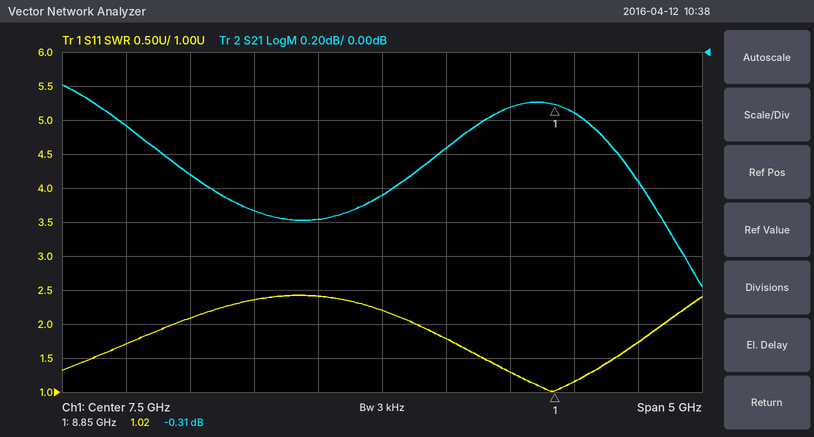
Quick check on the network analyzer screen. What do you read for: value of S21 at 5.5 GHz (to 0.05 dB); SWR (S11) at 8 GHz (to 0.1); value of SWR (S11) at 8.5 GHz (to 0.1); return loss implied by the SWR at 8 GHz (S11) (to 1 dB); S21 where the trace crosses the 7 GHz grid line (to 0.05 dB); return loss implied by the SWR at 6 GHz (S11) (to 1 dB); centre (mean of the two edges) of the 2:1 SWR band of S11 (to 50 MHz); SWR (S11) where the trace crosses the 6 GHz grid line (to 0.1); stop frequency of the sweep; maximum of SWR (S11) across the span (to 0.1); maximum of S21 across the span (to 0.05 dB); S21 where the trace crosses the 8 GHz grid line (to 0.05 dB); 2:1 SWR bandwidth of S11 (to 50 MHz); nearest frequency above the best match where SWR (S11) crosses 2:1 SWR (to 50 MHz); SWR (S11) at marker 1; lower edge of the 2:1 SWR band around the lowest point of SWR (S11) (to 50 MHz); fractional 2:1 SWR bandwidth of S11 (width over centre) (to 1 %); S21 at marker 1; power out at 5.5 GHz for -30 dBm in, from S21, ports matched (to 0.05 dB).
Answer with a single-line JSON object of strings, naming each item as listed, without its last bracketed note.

{"value of S21 at 5.5 GHz": "-0.45 dB", "SWR (S11) at 8 GHz": "1.8", "value of SWR (S11) at 8.5 GHz": "1.3", "return loss implied by the SWR at 8 GHz (S11)": "11 dB", "S21 where the trace crosses the 7 GHz grid line": "-1.00 dB", "return loss implied by the SWR at 6 GHz (S11)": "9 dB", "centre (mean of the two edges) of the 2:1 SWR band of S11": "8.75 GHz", "SWR (S11) where the trace crosses the 6 GHz grid line": "2.1", "stop frequency of the sweep": "10 GHz", "maximum of SWR (S11) across the span": "2.4", "maximum of S21 across the span": "-0.20 dB", "S21 where the trace crosses the 8 GHz grid line": "-0.55 dB", "2:1 SWR bandwidth of S11": "1.95 GHz", "nearest frequency above the best match where SWR (S11) crosses 2:1 SWR": "9.70 GHz", "SWR (S11) at marker 1": "1.02", "lower edge of the 2:1 SWR band around the lowest point of SWR (S11)": "7.75 GHz", "fractional 2:1 SWR bandwidth of S11 (width over centre)": "22 %", "S21 at marker 1": "-0.31 dB", "power out at 5.5 GHz for -30 dBm in, from S21, ports matched": "-30.45 dBm"}
